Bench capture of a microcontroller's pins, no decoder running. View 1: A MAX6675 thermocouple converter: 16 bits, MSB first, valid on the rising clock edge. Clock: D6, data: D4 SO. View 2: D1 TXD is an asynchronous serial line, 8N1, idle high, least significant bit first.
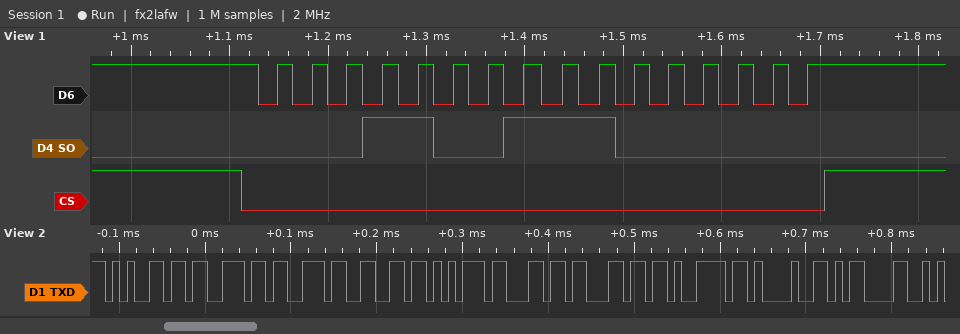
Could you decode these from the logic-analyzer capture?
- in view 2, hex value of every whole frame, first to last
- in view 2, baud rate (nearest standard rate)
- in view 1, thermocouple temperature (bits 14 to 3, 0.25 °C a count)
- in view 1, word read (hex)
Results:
65 73 73 66 75 6C 6C 79 21 0D
115200 baud
206.00 °C
0x19C0
